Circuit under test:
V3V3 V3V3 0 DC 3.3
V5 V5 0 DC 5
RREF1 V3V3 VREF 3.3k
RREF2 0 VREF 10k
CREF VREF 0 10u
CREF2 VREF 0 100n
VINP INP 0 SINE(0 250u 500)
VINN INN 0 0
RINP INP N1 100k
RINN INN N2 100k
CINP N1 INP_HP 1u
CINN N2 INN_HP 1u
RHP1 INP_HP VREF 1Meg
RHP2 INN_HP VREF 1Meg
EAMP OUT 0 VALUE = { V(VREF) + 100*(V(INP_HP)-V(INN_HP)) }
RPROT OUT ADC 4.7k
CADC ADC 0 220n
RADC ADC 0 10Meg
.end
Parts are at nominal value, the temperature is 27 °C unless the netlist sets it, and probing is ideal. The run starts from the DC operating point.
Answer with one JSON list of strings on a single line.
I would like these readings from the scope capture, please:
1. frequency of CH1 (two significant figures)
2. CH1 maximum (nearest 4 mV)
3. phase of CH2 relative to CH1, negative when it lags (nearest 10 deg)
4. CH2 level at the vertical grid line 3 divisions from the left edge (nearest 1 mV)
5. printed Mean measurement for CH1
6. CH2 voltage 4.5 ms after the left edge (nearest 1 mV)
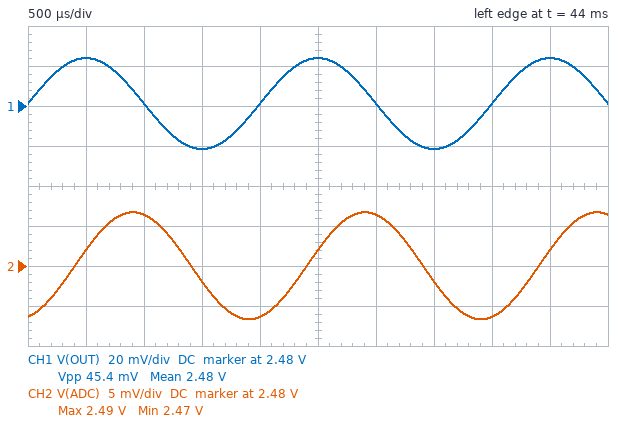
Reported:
["500 Hz", "2.504 V", "-70 deg", "2.478 V", "2.48 V", "2.482 V"]
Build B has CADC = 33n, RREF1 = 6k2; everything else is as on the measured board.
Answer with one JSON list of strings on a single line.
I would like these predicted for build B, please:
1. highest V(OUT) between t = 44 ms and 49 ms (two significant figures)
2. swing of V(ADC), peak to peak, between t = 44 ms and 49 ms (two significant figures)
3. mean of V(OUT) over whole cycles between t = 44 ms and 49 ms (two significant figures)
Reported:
["2.1 V", "41 mV", "2.0 V"]
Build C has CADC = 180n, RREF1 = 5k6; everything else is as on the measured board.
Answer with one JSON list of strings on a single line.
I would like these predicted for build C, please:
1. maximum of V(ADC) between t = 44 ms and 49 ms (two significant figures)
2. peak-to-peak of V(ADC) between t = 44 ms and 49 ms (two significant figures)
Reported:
["2.1 V", "16 mV"]
